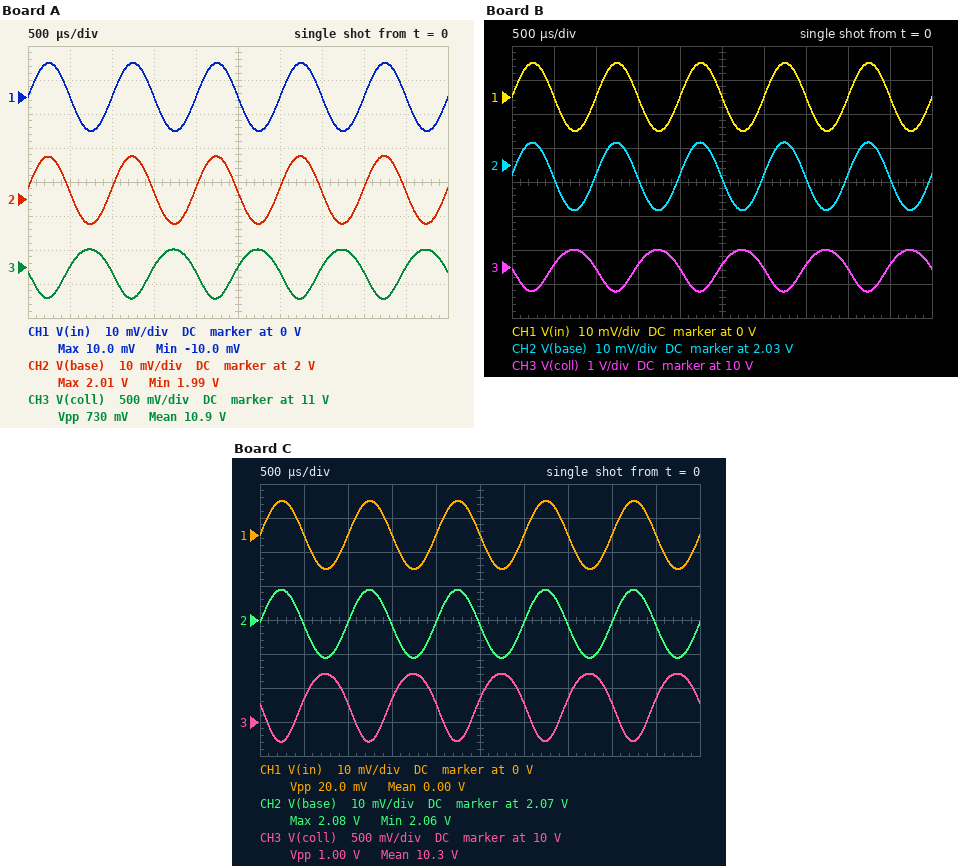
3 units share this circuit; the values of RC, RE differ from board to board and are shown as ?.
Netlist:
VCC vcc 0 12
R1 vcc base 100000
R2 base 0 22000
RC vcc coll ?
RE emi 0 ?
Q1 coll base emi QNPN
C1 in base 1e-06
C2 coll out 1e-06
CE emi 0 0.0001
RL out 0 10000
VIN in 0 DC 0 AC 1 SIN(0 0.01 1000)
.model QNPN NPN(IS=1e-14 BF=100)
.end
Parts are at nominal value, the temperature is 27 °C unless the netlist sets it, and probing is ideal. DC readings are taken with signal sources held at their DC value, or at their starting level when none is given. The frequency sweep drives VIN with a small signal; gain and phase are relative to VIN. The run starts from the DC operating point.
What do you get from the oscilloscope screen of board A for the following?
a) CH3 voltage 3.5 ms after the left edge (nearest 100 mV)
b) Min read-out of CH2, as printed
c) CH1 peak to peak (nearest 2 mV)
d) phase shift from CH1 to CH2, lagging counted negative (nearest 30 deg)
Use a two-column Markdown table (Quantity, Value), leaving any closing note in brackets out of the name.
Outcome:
| Quantity | Value |
|---|---|
| CH3 voltage 3.5 ms after the left edge | 11.0 V |
| Min read-out of CH2, as printed | 1.99 V |
| CH1 peak to peak | 20 mV |
| phase shift from CH1 to CH2, lagging counted negative | 0 deg |
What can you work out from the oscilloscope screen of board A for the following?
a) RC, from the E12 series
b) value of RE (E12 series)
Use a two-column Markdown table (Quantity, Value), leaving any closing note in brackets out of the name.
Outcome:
| Quantity | Value |
|---|---|
| RC, from the E12 series | 1.2 kΩ |
| value of RE | 1.5 kΩ |
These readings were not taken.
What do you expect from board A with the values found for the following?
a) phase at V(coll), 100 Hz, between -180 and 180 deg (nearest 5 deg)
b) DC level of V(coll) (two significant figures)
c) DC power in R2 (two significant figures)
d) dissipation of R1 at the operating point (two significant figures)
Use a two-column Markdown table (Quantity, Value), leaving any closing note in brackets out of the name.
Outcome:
| Quantity | Value |
|---|---|
| phase at V(coll), 100 Hz, between -180 and 180 deg | -130 deg |
| DC level of V(coll) | 11 V |
| DC power in R2 | 180 µW |
| dissipation of R1 at the operating point | 1.0 mW |
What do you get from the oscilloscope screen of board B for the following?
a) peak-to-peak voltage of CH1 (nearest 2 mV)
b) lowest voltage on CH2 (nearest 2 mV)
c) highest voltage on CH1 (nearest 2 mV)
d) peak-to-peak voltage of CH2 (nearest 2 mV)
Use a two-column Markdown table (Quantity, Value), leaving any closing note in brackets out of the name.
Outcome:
| Quantity | Value |
|---|---|
| peak-to-peak voltage of CH1 | 20 mV |
| lowest voltage on CH2 | 2.016 V |
| highest voltage on CH1 | 10 mV |
| peak-to-peak voltage of CH2 | 20 mV |
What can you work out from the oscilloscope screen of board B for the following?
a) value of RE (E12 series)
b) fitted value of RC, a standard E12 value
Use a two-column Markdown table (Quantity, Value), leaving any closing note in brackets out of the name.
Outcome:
| Quantity | Value |
|---|---|
| value of RE | 1.8 kΩ |
| fitted value of RC, a standard E12 value | 2.7 kΩ |
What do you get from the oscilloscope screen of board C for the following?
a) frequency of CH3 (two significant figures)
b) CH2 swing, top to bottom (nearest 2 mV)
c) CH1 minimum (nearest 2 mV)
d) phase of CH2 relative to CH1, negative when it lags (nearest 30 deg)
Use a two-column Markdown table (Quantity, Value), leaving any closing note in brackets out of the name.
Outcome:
| Quantity | Value |
|---|---|
| frequency of CH3 | 1.0 kHz |
| CH2 swing, top to bottom | 20 mV |
| CH1 minimum | -10 mV |
| phase of CH2 relative to CH1, negative when it lags | 0 deg |
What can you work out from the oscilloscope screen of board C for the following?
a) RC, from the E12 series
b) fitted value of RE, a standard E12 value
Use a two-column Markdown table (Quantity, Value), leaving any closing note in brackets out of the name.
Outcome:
| Quantity | Value |
|---|---|
| RC, from the E12 series | 3.3 kΩ |
| fitted value of RE, a standard E12 value | 2.7 kΩ |
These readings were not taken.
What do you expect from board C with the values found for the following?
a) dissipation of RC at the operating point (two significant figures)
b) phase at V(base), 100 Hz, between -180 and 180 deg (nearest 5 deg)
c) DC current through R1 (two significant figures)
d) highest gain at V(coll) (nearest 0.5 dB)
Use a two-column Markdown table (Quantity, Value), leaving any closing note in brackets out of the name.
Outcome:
| Quantity | Value |
|---|---|
| dissipation of RC at the operating point | 910 µW |
| phase at V(base), 100 Hz, between -180 and 180 deg | 20 deg |
| DC current through R1 | 99 µA |
| highest gain at V(coll) | 34.0 dB |
